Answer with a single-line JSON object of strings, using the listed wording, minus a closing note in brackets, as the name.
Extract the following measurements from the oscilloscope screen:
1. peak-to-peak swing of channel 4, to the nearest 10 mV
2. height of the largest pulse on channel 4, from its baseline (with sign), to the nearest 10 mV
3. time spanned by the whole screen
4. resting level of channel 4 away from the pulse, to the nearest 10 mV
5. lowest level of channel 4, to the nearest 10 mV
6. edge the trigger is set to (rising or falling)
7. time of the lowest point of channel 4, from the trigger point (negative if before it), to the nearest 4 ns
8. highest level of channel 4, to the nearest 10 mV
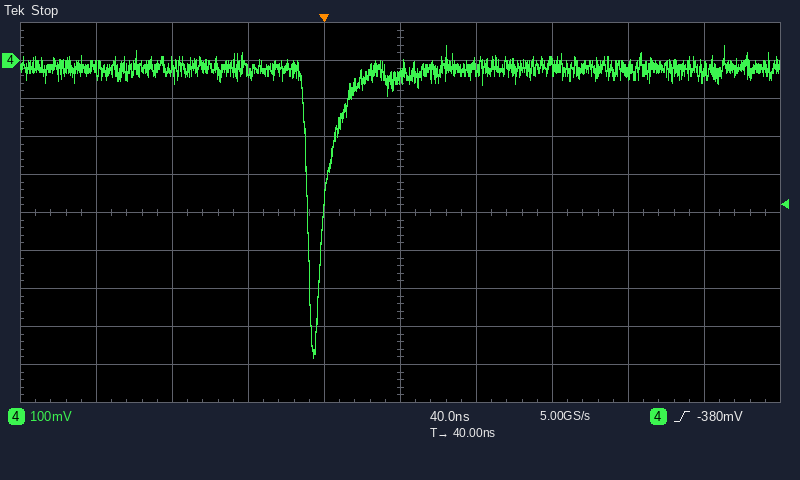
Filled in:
{"peak-to-peak swing of channel 4, to the nearest 10 mV": "820 mV", "height of the largest pulse on channel 4, from its baseline (with sign), to the nearest 10 mV": "-760 mV", "time spanned by the whole screen": "400 ns", "resting level of channel 4 away from the pulse, to the nearest 10 mV": "-20 mV", "lowest level of channel 4, to the nearest 10 mV": "-780 mV", "edge the trigger is set to": "rising", "time of the lowest point of channel 4, from the trigger point (negative if before it), to the nearest 4 ns": "-4 ns", "highest level of channel 4, to the nearest 10 mV": "40 mV"}
